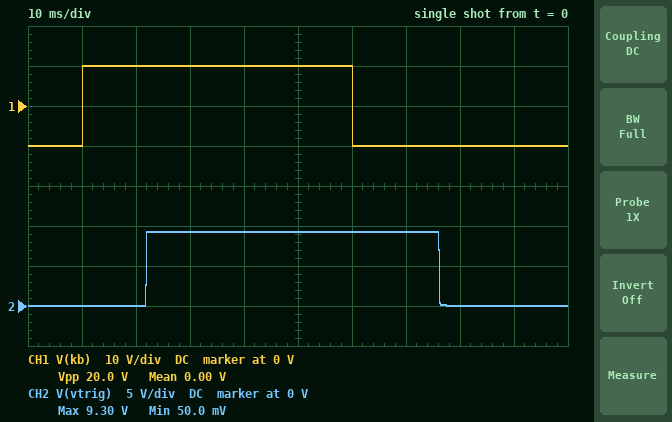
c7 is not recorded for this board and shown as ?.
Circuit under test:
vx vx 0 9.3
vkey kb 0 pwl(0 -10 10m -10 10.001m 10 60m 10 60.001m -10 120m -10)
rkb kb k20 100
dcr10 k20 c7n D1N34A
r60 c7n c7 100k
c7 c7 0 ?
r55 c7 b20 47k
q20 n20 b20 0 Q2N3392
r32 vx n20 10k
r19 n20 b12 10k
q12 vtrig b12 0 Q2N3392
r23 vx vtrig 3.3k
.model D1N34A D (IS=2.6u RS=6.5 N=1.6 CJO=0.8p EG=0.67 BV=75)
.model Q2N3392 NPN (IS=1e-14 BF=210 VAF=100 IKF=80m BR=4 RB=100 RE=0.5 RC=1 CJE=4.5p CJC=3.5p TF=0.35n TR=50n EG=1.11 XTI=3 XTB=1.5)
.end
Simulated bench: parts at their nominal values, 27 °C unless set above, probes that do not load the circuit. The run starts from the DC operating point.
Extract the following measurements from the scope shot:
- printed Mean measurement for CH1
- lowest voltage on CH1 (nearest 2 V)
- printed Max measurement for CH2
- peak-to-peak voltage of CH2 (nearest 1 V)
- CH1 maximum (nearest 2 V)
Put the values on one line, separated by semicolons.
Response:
0.00 V; -10 V; 9.30 V; 9 V; 10 V
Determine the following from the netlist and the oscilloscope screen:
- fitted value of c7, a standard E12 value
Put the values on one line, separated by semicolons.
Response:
150 nF
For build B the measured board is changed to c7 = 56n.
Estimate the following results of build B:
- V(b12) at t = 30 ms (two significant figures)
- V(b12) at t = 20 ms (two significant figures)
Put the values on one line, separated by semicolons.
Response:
45 mV; 46 mV
